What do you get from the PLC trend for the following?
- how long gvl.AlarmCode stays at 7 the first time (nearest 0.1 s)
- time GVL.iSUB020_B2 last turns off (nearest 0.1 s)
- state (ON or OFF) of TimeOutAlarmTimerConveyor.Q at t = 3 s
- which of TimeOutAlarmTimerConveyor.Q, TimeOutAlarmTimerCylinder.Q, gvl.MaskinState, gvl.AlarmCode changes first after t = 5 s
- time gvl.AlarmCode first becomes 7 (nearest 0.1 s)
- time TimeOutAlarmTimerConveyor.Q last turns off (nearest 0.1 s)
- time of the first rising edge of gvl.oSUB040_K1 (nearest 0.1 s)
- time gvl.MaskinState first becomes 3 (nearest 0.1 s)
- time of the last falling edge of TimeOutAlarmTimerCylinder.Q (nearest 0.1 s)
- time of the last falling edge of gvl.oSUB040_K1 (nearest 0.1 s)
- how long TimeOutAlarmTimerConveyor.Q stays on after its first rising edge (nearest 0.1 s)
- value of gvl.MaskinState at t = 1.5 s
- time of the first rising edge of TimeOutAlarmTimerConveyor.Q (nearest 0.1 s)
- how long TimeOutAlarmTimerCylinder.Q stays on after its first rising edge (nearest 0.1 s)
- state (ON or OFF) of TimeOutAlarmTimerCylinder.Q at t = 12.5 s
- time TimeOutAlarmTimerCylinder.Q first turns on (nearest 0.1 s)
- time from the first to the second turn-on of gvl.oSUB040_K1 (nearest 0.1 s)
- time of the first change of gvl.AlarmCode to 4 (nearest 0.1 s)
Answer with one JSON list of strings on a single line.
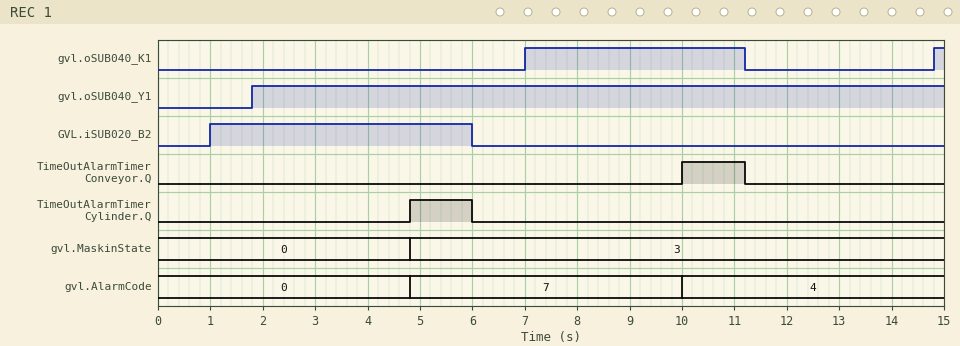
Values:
["5.2 s", "6.0 s", "OFF", "TimeOutAlarmTimerCylinder.Q", "4.8 s", "11.2 s", "7.0 s", "4.8 s", "6.0 s", "11.2 s", "1.2 s", "0", "10.0 s", "1.2 s", "OFF", "4.8 s", "7.8 s", "10.0 s"]
